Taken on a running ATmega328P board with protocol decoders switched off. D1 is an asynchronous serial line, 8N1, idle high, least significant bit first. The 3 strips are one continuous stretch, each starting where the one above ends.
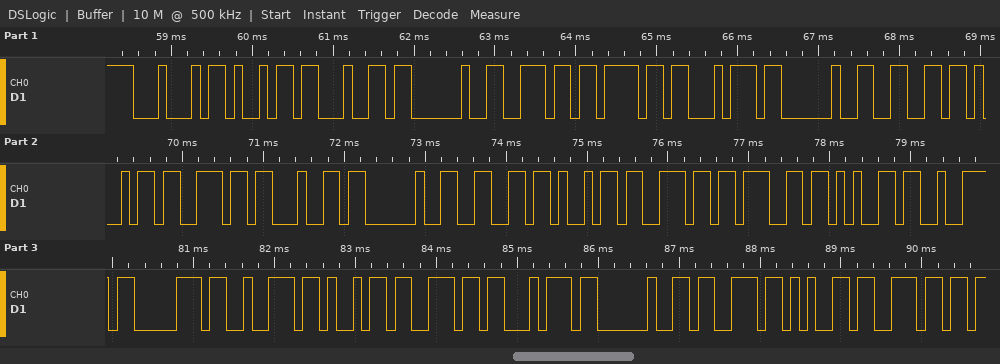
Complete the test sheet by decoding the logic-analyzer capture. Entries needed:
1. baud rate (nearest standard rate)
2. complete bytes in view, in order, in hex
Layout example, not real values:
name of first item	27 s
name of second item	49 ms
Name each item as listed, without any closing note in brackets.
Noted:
baud rate	9600 baud
complete bytes in view, in order, in hex	44 69 64 20 6E 6F 74 20 66 69 6E 64 20 66 69 6E 67 65 72 70 72 69 6E 74 20 73 65 6E
